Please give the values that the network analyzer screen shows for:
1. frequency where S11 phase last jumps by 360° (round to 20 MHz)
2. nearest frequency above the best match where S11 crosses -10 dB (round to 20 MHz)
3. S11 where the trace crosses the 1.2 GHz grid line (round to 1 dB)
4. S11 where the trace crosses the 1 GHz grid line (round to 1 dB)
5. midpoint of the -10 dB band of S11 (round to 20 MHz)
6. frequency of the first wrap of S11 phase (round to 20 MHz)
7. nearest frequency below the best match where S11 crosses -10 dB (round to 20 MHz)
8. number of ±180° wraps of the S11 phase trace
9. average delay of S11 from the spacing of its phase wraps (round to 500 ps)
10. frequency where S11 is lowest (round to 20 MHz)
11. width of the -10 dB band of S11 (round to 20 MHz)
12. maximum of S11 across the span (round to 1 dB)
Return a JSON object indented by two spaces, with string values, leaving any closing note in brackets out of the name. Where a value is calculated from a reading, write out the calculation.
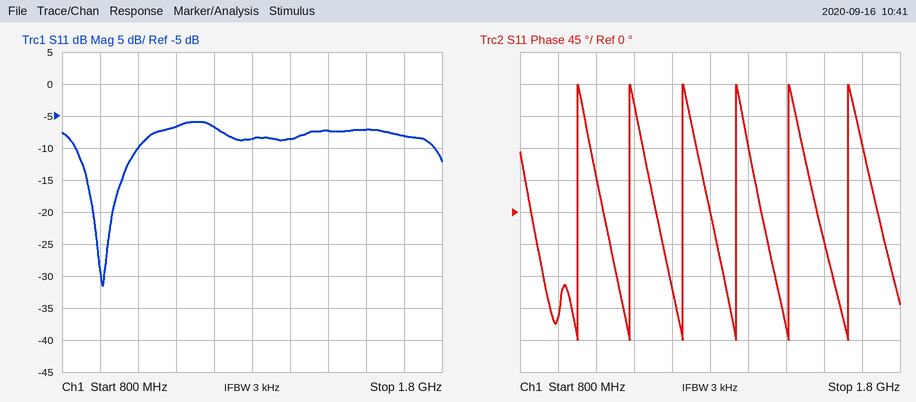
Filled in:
{
  "frequency where S11 phase last jumps by 360°": "1.66 GHz",
  "nearest frequency above the best match where S11 crosses -10 dB": "1.00 GHz",
  "S11 where the trace crosses the 1.2 GHz grid line": "-7 dB",
  "S11 where the trace crosses the 1 GHz grid line": "-10 dB",
  "midpoint of the -10 dB band of S11": "920 MHz",
  "frequency of the first wrap of S11 phase": "960 MHz",
  "nearest frequency below the best match where S11 crosses -10 dB": "840 MHz",
  "number of ±180° wraps of the S11 phase trace": "6",
  "average delay of S11 from the spacing of its phase wraps": "5 cycles / (1.66 GHz − 960 MHz) ≈ 7.14 ns, so 7.0 ns to the nearest 500 ps",
  "frequency where S11 is lowest": "900 MHz",
  "width of the -10 dB band of S11": "1.00 GHz − 840 MHz = 160 MHz",
  "maximum of S11 across the span": "-6 dB"
}
